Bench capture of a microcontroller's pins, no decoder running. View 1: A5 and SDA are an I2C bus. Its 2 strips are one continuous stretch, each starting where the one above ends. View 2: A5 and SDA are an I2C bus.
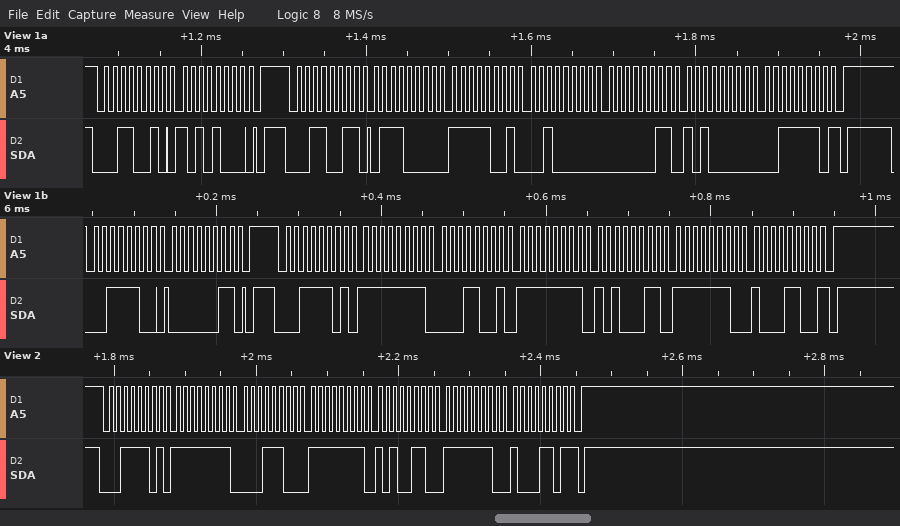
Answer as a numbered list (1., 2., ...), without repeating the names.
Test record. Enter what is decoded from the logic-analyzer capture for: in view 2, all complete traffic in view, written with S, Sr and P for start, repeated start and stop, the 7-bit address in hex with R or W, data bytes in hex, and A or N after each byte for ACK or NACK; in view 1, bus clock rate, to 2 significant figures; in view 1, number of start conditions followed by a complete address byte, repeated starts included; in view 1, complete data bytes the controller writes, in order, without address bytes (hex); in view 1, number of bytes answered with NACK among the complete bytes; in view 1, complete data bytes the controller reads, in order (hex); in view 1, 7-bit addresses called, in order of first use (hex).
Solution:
1. S 1ER A FF A 1C A FF A A6 A FE A 8D N P
2. 100 kHz
3. 4
4. A8 03
5. 2
6. 70 F9 20 03 A0 3E FF 19 FF A3 FE 8C
7. 0x19 0x1E
